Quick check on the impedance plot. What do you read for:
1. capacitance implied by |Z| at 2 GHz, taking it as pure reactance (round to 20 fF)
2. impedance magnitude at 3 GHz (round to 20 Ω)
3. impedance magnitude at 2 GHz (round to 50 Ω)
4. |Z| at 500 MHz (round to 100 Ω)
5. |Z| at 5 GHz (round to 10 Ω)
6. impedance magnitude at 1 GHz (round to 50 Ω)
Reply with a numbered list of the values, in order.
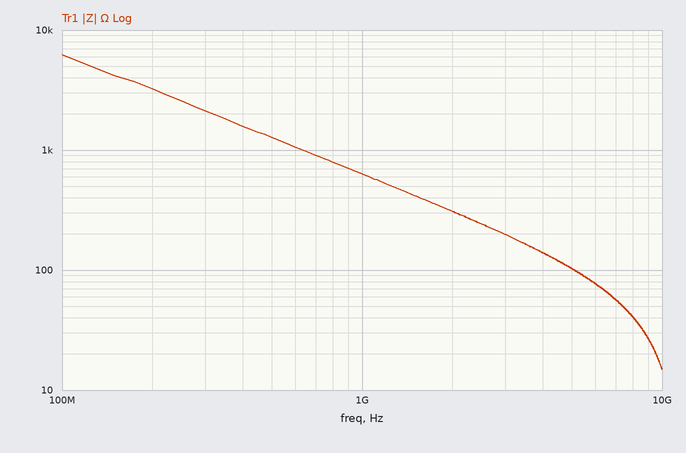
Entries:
1. 260 fF
2. 200 Ω
3. 300 Ω
4. 1.3 kΩ
5. 100 Ω
6. 650 Ω
